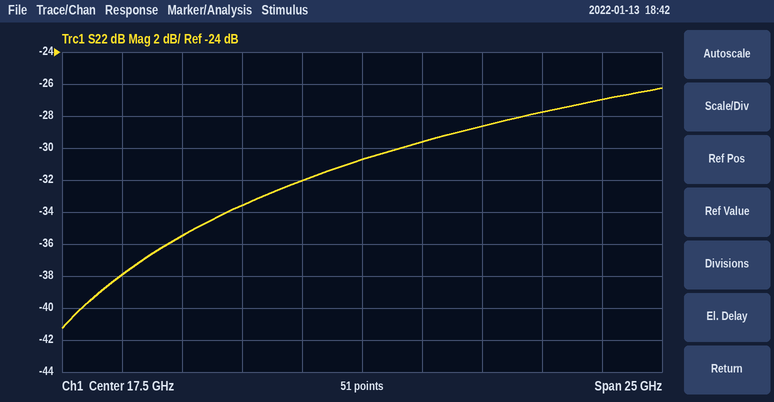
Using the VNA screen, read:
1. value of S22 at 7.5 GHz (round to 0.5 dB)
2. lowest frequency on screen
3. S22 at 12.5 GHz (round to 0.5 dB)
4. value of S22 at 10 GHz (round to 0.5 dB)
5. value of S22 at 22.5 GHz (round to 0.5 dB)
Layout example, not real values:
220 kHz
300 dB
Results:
-38.0 dB
5 GHz
-33.5 dB
-35.5 dB
-28.5 dB
